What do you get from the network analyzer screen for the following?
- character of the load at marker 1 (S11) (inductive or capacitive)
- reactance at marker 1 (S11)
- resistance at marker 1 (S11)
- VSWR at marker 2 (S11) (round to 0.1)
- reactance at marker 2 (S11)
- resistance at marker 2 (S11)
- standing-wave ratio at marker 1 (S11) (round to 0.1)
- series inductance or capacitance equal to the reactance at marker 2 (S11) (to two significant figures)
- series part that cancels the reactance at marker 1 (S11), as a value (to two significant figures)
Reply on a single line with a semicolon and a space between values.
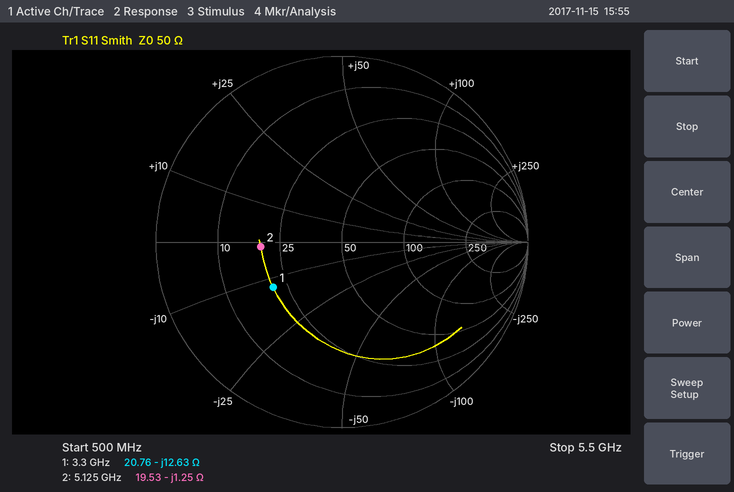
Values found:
capacitive; -12.63 Ω; 20.76 Ω; 2.6; -1.25 Ω; 19.53 Ω; 2.6; 25 pF; 610 pH
